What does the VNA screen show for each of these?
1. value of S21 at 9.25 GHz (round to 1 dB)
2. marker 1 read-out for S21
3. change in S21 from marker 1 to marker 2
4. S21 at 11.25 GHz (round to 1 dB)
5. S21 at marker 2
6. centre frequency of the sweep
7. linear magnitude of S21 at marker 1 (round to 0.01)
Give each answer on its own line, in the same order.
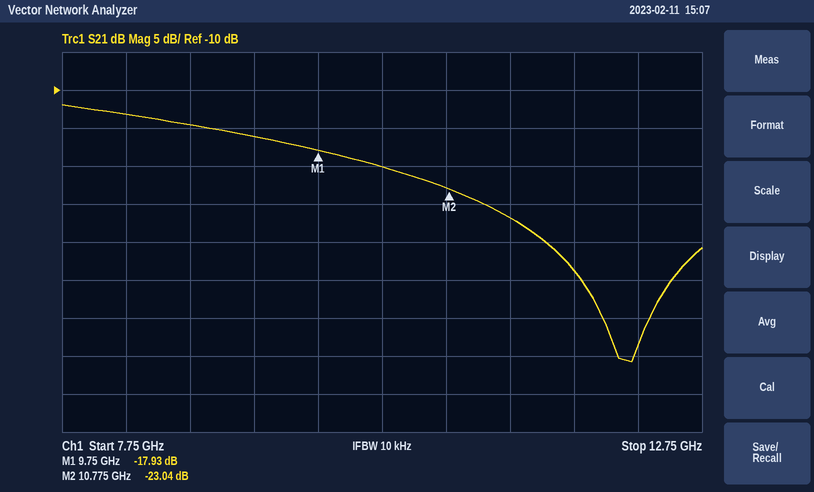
-16 dB
-17.93 dB
-5.11 dB
-27 dB
-23.04 dB
10.25 GHz
0.13
